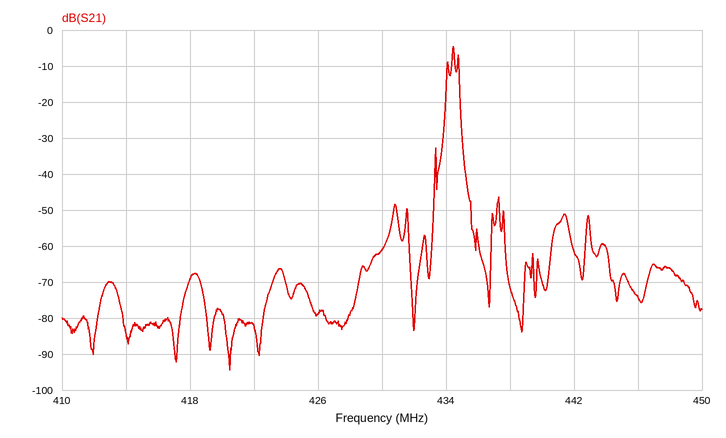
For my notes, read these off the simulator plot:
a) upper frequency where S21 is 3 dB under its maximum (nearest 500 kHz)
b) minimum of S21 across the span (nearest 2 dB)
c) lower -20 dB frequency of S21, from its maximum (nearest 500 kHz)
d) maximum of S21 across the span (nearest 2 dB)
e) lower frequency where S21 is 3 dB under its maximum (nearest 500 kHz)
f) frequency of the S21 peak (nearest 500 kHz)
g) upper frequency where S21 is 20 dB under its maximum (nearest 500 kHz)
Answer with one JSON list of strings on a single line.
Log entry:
["434.5 MHz", "-94 dB", "434.0 MHz", "-4 dB", "434.5 MHz", "434.5 MHz", "435.0 MHz"]
